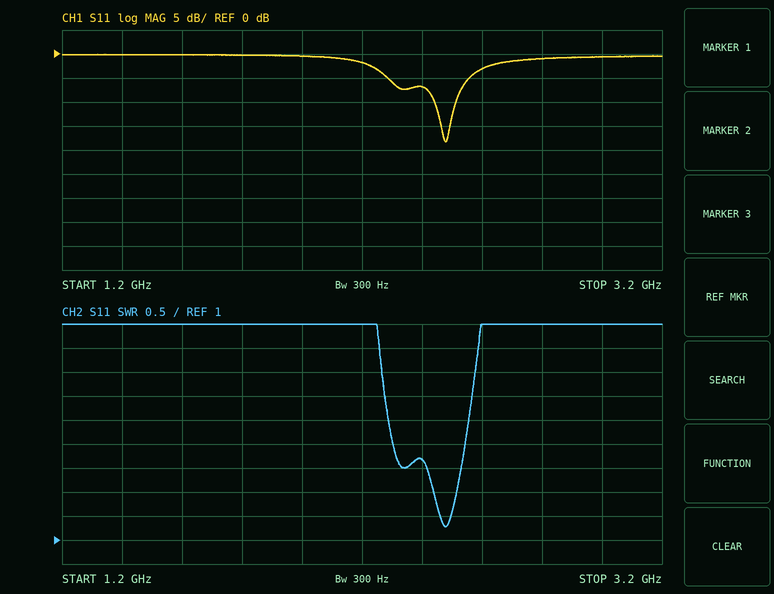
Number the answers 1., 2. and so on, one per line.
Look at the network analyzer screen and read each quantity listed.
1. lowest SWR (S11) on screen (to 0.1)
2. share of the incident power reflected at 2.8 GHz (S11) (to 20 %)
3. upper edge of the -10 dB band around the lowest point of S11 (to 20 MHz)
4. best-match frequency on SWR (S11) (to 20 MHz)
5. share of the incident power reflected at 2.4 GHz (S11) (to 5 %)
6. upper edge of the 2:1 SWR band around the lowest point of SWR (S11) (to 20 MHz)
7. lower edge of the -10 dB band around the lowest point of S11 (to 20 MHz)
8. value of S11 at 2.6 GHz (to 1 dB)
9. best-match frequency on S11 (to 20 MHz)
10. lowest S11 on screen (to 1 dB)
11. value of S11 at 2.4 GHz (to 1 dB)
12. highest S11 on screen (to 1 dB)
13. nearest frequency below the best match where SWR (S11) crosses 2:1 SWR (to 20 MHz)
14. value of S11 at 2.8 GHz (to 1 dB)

1. 1.3
2. 80 %
3. 2.52 GHz
4. 2.48 GHz
5. 20 %
6. 2.52 GHz
7. 2.44 GHz
8. -3 dB
9. 2.48 GHz
10. -18 dB
11. -7 dB
12. 0 dB
13. 2.44 GHz
14. -1 dB
